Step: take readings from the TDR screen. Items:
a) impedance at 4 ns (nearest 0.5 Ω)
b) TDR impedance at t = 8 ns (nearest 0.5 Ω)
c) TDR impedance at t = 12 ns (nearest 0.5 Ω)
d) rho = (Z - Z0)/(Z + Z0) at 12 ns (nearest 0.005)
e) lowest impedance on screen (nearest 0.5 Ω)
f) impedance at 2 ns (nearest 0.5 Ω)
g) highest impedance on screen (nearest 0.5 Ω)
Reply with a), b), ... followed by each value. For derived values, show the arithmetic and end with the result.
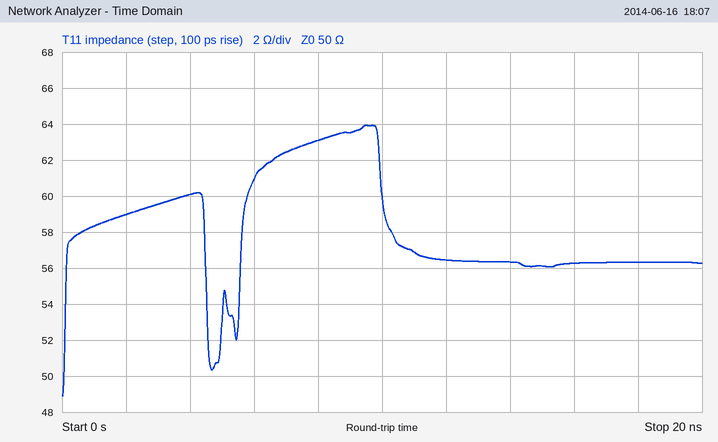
a) 60.0 Ω
b) 63.0 Ω
c) 56.5 Ω
d) (56.5 − 50)/(56.5 + 50) ≈ +0.0610, so +0.060 to the nearest 0.005
e) 49.0 Ω
f) 59.0 Ω
g) 64.0 Ω
